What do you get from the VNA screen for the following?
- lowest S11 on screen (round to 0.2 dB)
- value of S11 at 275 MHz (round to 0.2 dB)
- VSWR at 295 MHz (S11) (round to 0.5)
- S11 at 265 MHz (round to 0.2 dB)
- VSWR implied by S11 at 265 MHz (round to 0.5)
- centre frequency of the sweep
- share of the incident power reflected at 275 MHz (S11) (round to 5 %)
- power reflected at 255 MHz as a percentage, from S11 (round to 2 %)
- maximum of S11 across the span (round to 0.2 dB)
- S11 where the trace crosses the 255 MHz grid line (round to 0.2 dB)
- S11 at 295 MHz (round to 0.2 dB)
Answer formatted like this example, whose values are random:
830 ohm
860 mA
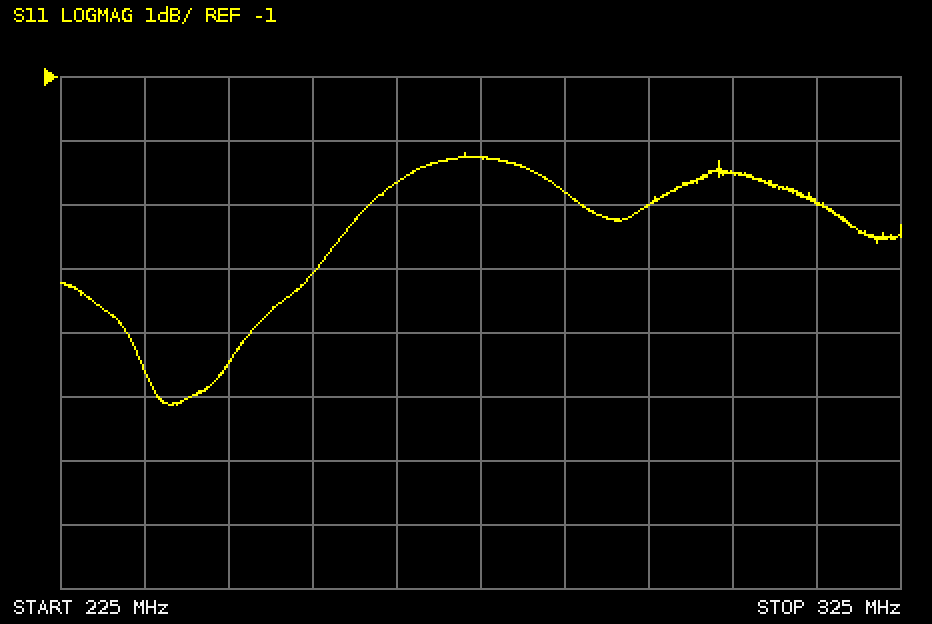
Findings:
-6.2 dB
-2.2 dB
6.0
-2.6 dB
6.5
275 MHz
60 %
40 %
-2.2 dB
-4.0 dB
-3.0 dB
